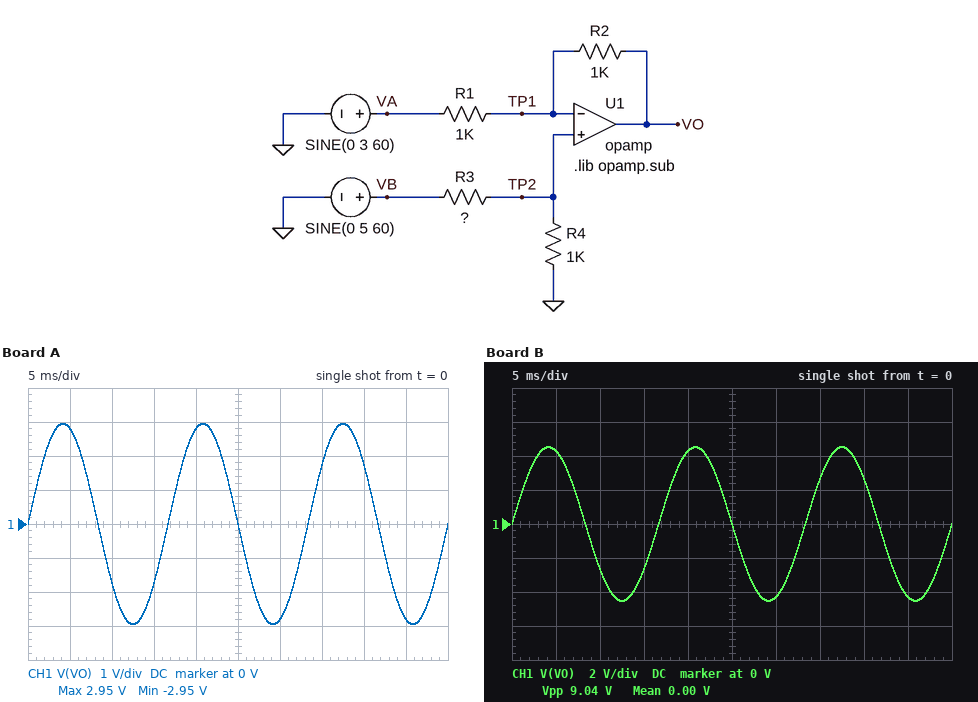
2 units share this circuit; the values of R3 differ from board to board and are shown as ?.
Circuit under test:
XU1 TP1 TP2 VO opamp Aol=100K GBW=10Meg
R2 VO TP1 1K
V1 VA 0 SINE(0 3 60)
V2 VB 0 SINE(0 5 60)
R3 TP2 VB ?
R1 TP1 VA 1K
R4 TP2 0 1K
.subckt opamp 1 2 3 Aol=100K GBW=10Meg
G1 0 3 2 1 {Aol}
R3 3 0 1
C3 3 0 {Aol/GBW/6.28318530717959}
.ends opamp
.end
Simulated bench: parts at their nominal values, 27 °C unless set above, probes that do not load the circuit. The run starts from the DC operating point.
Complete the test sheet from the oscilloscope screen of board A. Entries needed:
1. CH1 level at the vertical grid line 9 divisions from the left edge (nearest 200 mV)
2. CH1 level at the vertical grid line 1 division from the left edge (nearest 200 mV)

-2.8 V
2.8 V
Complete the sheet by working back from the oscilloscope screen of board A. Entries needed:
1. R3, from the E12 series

680 Ω
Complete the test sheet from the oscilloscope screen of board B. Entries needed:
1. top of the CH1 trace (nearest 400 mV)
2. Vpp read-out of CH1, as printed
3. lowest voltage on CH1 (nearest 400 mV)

4.4 V
9.04 V
-4.4 V
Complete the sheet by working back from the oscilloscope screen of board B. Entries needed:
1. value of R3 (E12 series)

330 Ω
